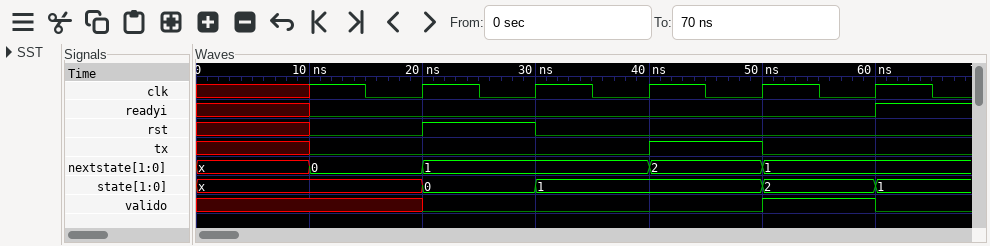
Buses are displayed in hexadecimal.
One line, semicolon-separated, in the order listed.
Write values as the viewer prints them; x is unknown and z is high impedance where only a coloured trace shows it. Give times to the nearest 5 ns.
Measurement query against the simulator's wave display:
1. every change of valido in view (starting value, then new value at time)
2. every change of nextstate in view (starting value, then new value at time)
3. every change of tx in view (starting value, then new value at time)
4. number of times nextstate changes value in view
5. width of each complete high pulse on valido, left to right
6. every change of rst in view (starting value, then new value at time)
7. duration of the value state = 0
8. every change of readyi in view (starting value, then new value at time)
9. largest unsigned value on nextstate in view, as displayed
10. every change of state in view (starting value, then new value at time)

x, 0 at 20 ns, 1 at 50 ns, 0 at 60 ns; x, 0 at 10 ns, 1 at 20 ns, 2 at 40 ns, 1 at 50 ns; x, 0 at 10 ns, 1 at 40 ns, 0 at 50 ns; 4; 10 ns; x, 0 at 10 ns, 1 at 20 ns, 0 at 30 ns; 10 ns; x, 0 at 10 ns, 1 at 60 ns; 2; x, 0 at 20 ns, 1 at 30 ns, 2 at 50 ns, 1 at 60 ns
